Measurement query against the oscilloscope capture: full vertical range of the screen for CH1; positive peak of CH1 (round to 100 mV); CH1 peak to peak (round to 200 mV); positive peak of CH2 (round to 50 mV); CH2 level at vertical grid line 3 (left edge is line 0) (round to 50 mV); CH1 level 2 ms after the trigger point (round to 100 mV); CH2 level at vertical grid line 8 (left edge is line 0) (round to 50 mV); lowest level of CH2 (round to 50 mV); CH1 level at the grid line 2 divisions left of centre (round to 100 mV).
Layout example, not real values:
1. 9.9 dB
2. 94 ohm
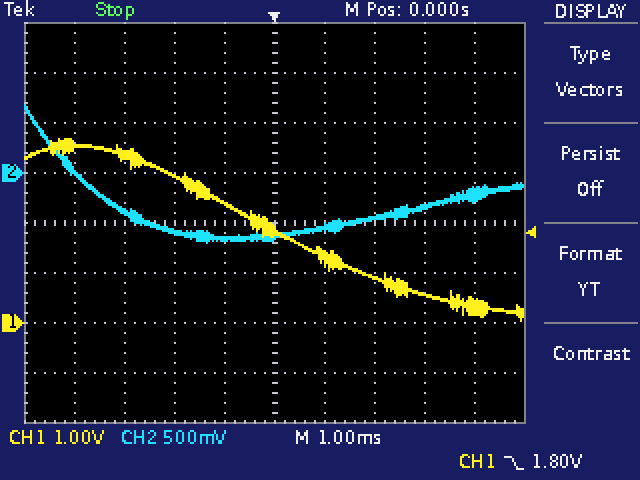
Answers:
1. 8 V
2. 3.7 V
3. 3.6 V
4. 700 mV
5. -600 mV
6. 900 mV
7. -350 mV
8. -700 mV
9. 2.9 V
